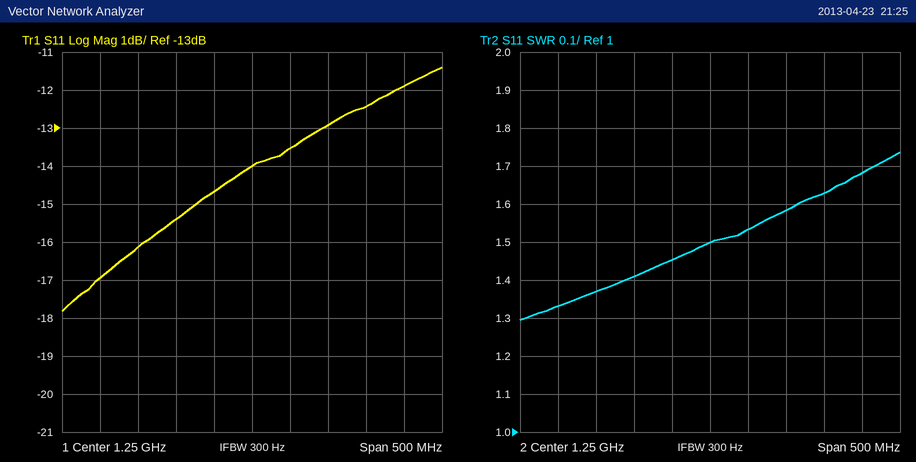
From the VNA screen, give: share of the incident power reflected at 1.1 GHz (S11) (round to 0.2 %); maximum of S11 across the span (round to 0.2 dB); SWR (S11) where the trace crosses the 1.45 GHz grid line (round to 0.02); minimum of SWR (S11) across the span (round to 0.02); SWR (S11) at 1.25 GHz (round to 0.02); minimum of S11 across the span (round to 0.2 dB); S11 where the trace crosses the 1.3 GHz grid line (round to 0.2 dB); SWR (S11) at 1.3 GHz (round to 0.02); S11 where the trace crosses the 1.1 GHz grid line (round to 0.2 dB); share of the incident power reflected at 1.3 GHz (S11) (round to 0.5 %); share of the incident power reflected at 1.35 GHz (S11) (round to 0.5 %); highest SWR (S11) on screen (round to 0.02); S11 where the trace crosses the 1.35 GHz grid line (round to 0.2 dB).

2.4 %
-11.4 dB
1.68
1.30
1.50
-17.8 dB
-13.6 dB
1.54
-16.2 dB
4.5 %
5.0 %
1.74
-13.0 dB
